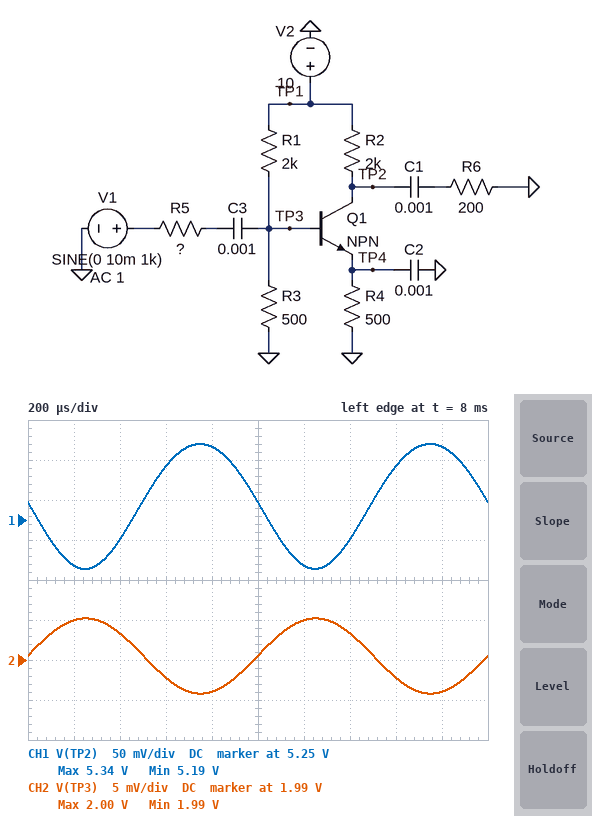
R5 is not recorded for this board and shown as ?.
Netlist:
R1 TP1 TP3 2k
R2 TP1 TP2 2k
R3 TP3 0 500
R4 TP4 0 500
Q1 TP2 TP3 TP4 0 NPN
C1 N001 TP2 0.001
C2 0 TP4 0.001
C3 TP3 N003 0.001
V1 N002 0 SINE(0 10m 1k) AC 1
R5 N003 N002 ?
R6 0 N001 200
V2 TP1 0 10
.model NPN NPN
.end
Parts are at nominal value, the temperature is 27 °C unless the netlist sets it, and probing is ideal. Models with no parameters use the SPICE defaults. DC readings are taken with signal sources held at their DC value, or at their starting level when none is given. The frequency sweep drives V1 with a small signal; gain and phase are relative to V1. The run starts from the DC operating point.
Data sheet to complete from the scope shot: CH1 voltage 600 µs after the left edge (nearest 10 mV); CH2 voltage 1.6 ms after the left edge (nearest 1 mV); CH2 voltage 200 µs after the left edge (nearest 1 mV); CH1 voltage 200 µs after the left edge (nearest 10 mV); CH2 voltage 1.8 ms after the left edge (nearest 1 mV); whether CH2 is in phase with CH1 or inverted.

5.32 V
1.988 V
1.995 V
5.19 V
1.986 V
inverted
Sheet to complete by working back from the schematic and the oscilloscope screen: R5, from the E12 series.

330 Ω
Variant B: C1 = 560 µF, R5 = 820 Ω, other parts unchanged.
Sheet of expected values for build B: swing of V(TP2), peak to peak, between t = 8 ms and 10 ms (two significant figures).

87 mV
